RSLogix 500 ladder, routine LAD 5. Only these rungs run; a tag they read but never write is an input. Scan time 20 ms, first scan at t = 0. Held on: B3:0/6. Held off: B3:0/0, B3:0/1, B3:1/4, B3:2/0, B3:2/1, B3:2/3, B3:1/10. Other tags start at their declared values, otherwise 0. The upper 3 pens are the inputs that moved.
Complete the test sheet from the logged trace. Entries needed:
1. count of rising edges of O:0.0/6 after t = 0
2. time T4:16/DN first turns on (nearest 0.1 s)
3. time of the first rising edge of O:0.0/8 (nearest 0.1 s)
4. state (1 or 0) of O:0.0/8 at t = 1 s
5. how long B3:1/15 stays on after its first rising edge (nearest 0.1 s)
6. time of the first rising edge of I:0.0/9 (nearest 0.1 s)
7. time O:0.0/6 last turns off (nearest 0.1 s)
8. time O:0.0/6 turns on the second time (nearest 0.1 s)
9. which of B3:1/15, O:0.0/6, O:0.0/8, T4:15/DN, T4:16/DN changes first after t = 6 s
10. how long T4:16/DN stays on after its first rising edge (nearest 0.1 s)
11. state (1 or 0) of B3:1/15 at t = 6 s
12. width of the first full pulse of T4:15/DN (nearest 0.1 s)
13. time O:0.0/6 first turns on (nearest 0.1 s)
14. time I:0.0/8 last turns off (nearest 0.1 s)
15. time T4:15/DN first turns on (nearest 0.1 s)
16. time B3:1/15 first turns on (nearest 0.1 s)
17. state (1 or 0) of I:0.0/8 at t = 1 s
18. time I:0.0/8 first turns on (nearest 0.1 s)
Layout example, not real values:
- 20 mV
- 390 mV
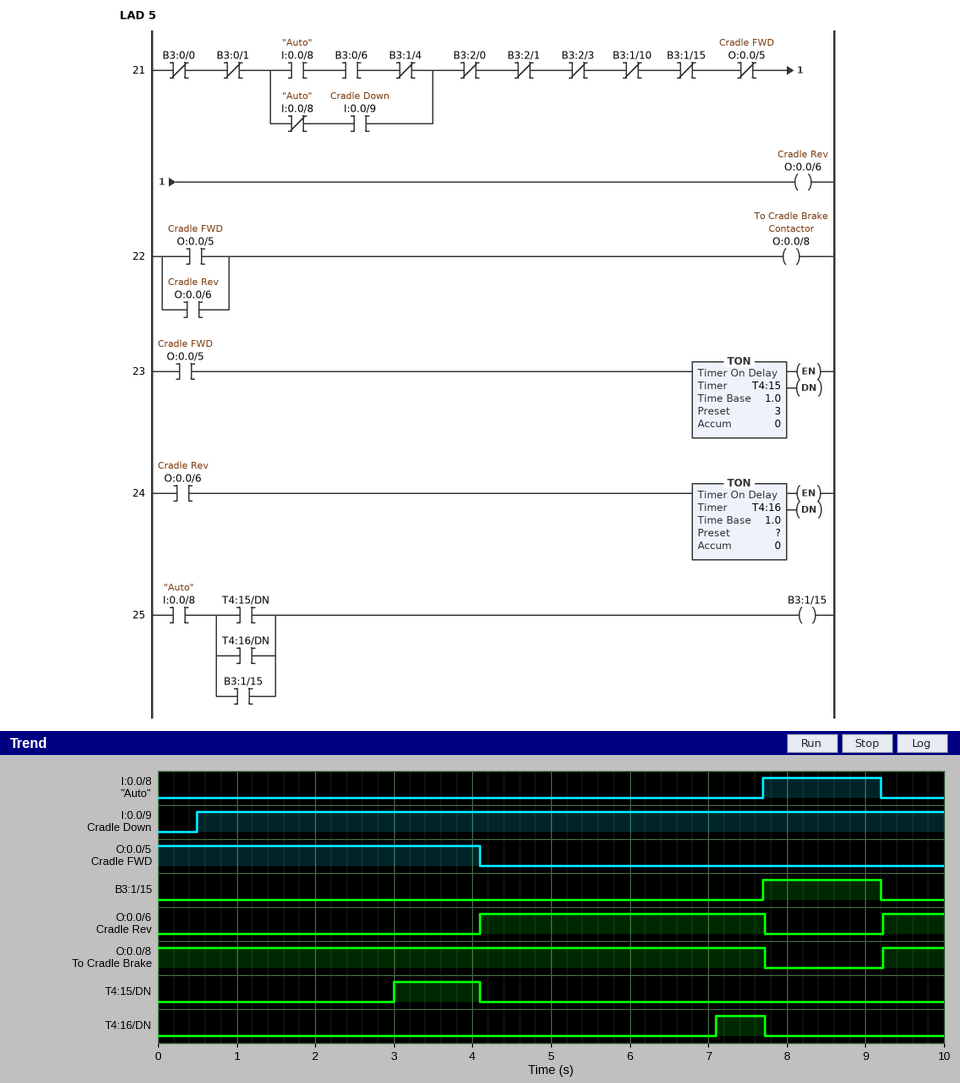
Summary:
- 2
- 7.1 s
- 9.2 s
- 1
- 1.5 s
- 0.5 s
- 7.7 s
- 9.2 s
- T4:16/DN
- 0.6 s
- 0
- 1.1 s
- 4.1 s
- 9.2 s
- 3.0 s
- 7.7 s
- 0
- 7.7 s
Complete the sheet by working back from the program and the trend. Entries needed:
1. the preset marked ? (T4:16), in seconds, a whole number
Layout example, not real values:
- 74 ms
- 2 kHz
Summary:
- 3 s
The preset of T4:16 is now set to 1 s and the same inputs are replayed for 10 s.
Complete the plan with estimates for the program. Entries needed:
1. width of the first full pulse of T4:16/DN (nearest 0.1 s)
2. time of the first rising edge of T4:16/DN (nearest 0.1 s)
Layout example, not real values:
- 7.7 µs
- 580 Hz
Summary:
- 2.6 s
- 5.1 s
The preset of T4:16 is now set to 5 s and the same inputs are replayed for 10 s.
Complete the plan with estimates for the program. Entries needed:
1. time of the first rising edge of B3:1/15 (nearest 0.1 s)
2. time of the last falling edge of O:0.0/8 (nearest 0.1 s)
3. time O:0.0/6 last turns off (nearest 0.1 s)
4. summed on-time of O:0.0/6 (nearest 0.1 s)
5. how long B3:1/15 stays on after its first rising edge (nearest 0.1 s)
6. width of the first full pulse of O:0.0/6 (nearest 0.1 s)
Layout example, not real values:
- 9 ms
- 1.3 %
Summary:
- 9.1 s
- 9.1 s
- 9.1 s
- 5.8 s
- 0.1 s
- 5.0 s
